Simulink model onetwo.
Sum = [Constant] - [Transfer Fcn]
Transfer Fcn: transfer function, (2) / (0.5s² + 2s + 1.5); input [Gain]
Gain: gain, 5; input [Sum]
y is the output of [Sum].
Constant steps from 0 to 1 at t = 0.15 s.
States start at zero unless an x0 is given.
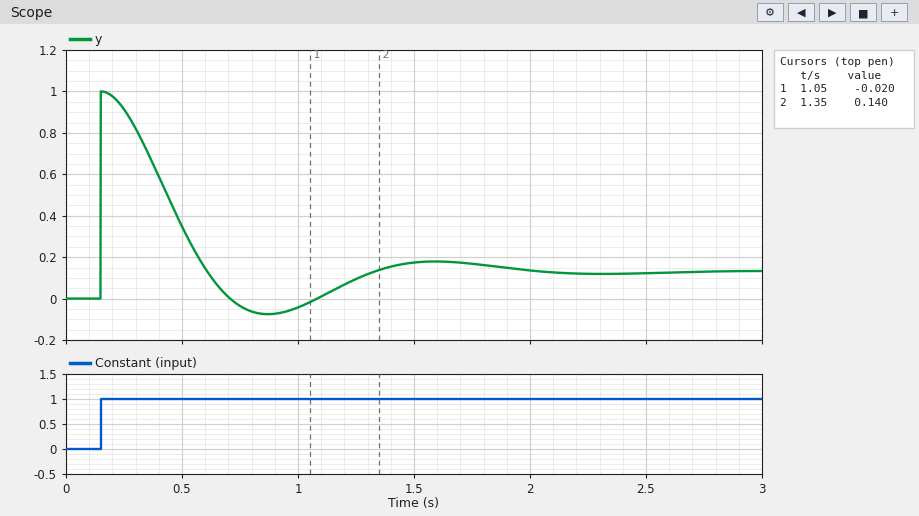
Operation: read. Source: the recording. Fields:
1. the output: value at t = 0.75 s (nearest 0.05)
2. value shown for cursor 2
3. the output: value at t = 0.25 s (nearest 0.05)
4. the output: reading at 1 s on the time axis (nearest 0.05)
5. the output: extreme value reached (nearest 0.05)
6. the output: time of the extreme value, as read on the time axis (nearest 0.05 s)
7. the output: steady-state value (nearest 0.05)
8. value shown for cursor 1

-0.05
0.140
0.90
-0.05
1.00
0.15 s
0.15
-0.020
